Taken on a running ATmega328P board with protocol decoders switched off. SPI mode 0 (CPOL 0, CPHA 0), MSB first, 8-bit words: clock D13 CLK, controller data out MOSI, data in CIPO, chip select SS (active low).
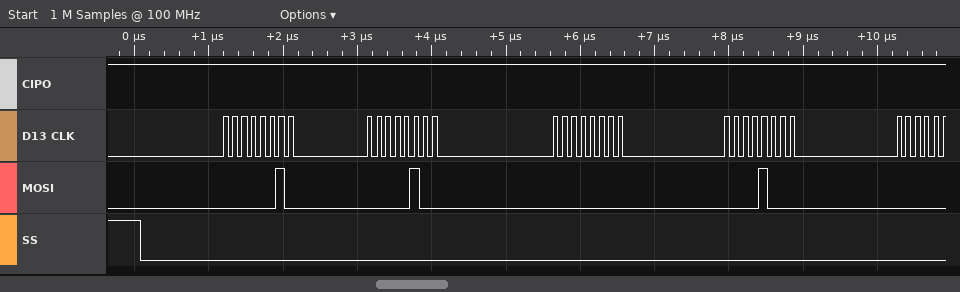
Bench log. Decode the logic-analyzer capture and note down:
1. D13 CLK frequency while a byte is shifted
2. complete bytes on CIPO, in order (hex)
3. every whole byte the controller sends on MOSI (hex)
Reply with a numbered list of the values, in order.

1. 8 MHz
2. 0xFF 0xFF 0xFF 0xFF
3. 0x02 0x04 0x00 0x08
